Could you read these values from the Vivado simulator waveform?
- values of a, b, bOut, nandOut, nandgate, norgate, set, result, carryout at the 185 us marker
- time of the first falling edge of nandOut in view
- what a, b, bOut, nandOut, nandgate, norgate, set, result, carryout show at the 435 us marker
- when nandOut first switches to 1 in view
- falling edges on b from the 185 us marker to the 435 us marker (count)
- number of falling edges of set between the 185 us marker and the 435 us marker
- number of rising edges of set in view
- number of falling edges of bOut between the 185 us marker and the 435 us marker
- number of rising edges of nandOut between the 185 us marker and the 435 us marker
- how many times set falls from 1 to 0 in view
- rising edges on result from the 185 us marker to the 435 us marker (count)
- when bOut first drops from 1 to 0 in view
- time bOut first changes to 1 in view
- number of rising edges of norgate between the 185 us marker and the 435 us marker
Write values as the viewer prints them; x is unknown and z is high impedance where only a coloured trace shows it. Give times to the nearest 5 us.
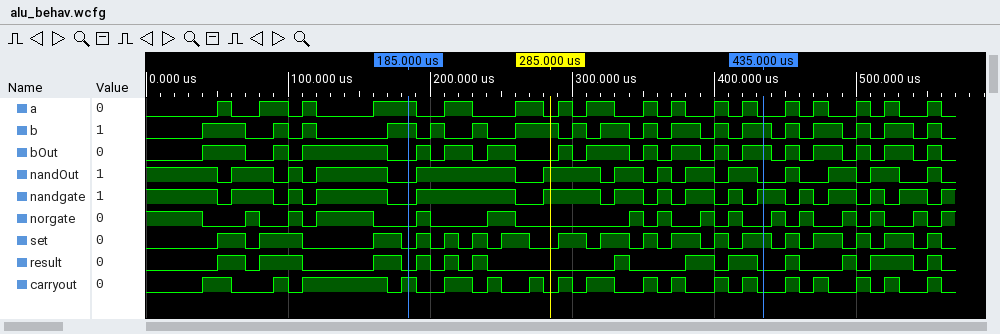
a=1, b=1, bOut=0, nandOut=0, nandgate=0, norgate=0, set=0, result=0, carryout=1
50 us
a=0, b=1, bOut=1, nandOut=0, nandgate=1, norgate=0, set=1, result=0, carryout=0
60 us
9
9
18
8
6
18
6
70 us
40 us
6
